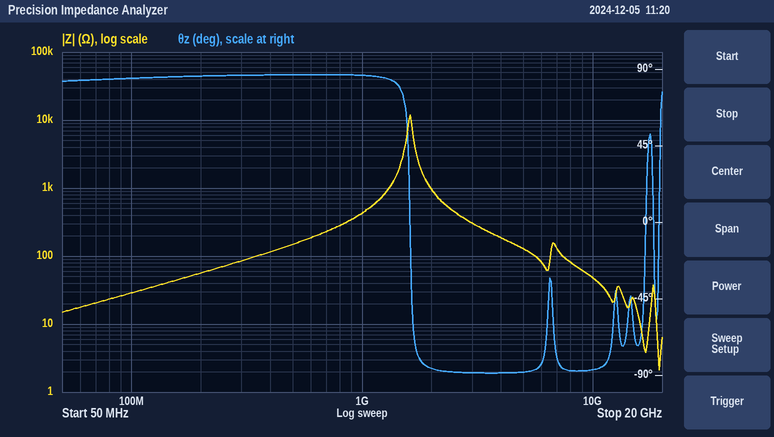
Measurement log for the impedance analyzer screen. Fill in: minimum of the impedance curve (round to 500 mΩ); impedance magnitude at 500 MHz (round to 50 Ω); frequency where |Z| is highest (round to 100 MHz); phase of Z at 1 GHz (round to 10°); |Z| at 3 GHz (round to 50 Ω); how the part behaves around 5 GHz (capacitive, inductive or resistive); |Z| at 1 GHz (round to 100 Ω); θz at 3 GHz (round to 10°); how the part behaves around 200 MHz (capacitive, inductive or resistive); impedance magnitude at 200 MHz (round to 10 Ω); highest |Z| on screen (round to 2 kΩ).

2.0 Ω
150 Ω
1.6 GHz
90°
300 Ω
capacitive
400 Ω
-90°
inductive
60 Ω
12 kΩ
